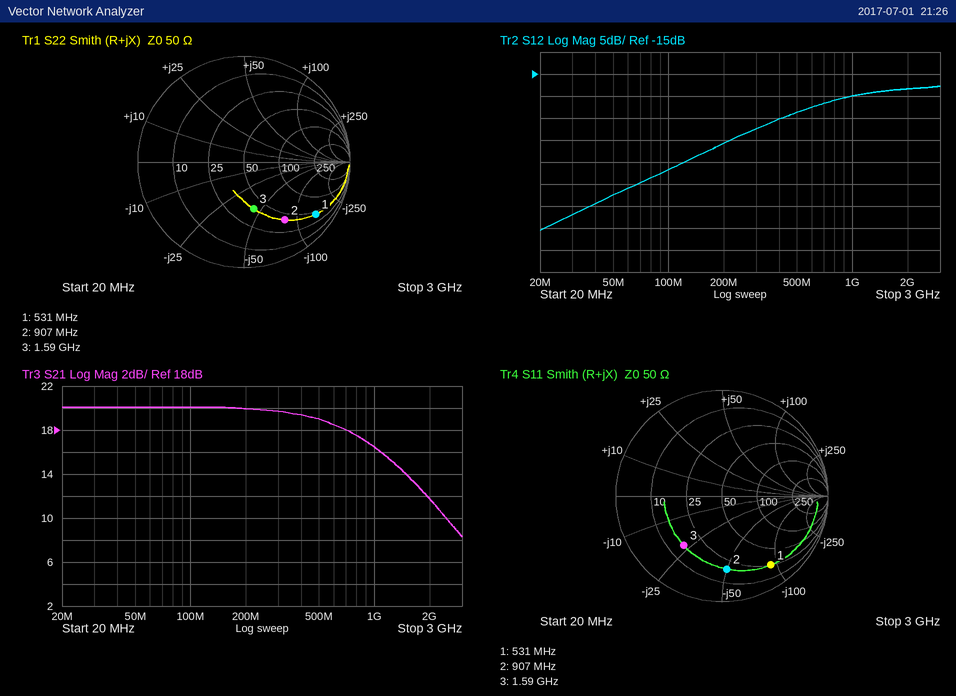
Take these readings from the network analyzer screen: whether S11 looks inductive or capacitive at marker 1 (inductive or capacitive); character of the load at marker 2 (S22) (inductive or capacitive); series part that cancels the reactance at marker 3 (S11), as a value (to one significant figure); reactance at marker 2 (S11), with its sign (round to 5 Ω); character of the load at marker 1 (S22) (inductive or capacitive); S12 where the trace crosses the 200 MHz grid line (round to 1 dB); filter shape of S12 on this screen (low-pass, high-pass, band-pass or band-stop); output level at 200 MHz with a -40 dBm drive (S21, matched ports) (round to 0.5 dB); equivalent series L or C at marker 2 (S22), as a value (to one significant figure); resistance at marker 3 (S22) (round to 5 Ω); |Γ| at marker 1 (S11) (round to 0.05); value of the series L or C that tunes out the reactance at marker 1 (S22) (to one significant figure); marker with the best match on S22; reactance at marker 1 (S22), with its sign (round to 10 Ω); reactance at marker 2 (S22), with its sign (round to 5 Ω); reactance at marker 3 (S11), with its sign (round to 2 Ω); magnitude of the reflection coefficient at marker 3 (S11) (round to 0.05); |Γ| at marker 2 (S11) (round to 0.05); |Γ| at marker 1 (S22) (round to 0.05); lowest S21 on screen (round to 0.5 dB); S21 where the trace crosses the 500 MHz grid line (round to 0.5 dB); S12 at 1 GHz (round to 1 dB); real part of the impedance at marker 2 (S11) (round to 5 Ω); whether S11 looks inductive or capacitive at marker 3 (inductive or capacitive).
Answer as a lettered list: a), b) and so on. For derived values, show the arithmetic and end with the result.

a) capacitive
b) capacitive
c) L = 22 Ω/(2π × 1.59 GHz) ≈ 2 nH
d) -50 Ω
e) capacitive
f) -31 dB
g) high-pass
h) -40 dBm + (20.0 dB) = -20.0 dBm
i) C = 1/(2π × 907 MHz × 80 Ω) ≈ 2 pF
j) 40 Ω
k) 0.80
l) L = 140 Ω/(2π × 531 MHz) ≈ 42.0 nH, so 40 nH to one significant figure
m) marker 3
n) -140 Ω
o) -80 Ω
p) -22 Ω
q) 0.60
r) 0.70
s) 0.85
t) 8.5 dB
u) 19.0 dB
v) -20 dB
w) 20 Ω
x) capacitive
